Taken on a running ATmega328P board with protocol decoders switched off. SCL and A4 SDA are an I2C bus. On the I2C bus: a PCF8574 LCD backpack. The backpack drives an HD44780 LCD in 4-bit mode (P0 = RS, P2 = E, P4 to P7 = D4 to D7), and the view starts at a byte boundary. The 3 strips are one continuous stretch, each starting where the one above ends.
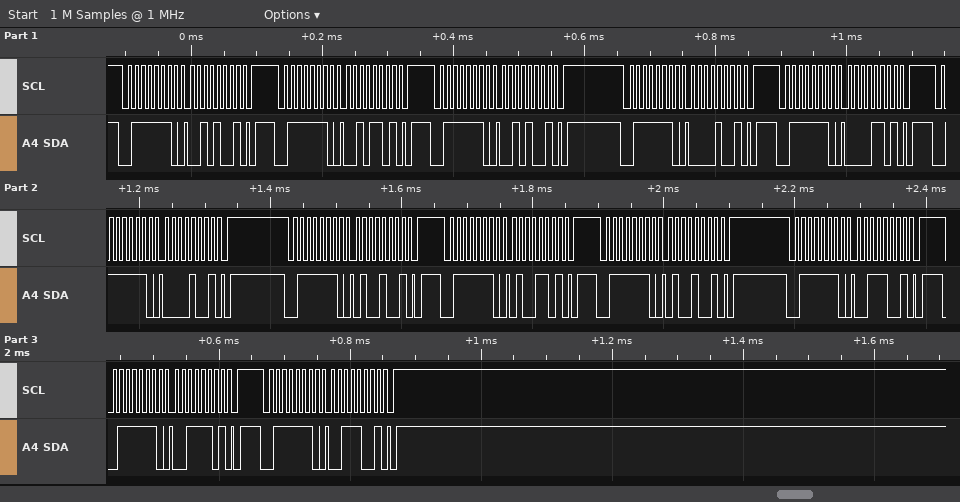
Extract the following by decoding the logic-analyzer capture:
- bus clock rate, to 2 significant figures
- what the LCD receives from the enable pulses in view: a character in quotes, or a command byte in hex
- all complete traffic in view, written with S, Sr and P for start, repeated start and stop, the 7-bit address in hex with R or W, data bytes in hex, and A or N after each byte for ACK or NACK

100 kHz
' ' 'C'
S 3FW A 29 A P S 3FW A 2D A P S 3FW A 29 A P S 3FW A 09 A P S 3FW A 0D A P S 3FW A 09 A P S 3FW A 49 A P S 3FW A 4D A P S 3FW A 49 A P S 3FW A 39 A P S 3FW A 3D A P S 3FW A 39 A P
